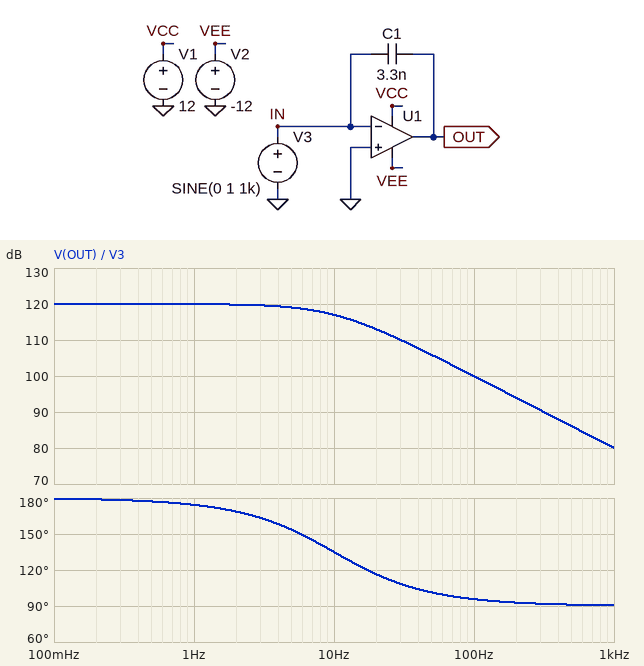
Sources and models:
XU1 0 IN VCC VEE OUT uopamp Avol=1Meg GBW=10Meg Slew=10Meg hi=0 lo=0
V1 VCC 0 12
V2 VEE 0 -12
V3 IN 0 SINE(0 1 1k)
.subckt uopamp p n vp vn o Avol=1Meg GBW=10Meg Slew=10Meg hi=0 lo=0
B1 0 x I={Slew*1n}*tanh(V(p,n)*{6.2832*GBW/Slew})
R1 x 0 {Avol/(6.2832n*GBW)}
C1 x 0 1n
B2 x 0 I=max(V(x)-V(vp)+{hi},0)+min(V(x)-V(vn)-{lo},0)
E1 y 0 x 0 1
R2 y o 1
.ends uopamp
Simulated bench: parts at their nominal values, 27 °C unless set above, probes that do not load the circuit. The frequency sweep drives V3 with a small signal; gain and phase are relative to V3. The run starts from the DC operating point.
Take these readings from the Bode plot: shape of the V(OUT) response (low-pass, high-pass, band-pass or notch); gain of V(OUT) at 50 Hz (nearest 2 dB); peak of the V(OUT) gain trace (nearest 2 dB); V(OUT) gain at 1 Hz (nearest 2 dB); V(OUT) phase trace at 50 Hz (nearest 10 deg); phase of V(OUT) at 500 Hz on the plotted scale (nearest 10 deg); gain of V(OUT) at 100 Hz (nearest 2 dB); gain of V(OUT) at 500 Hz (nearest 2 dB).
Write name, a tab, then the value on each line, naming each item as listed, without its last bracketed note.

shape of the V(OUT) response	low-pass
gain of V(OUT) at 50 Hz	106 dB
peak of the V(OUT) gain trace	120 dB
V(OUT) gain at 1 Hz	120 dB
V(OUT) phase trace at 50 Hz	100 deg
phase of V(OUT) at 500 Hz on the plotted scale	90 deg
gain of V(OUT) at 100 Hz	100 dB
gain of V(OUT) at 500 Hz	86 dB
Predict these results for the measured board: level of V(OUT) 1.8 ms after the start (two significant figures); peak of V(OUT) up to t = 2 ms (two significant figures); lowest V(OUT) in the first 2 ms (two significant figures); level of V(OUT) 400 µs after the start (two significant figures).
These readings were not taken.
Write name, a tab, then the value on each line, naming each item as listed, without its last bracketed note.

level of V(OUT) 1.8 ms after the start	12 V
peak of V(OUT) up to t = 2 ms	12 V
lowest V(OUT) in the first 2 ms	-12 V
level of V(OUT) 400 µs after the start	-12 V
